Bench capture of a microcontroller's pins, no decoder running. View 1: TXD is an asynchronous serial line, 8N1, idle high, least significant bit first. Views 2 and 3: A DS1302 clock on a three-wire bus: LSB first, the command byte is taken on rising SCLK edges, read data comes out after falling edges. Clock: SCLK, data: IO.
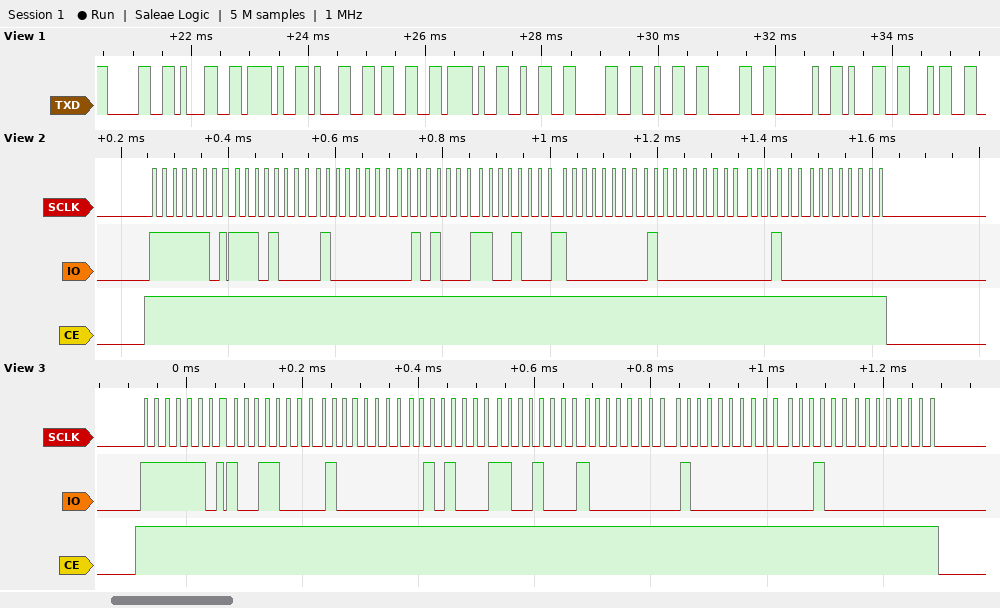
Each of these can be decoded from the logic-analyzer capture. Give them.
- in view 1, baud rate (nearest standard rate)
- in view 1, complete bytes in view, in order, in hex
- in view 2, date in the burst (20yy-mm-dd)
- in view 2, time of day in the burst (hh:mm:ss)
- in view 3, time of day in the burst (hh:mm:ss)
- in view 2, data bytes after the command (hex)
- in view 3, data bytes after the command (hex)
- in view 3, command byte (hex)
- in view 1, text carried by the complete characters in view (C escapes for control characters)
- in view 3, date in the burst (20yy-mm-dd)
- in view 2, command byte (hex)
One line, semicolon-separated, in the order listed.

9600 baud; 30 31 2F 31 33 2F 32 30 32 30 20 31 34; 2020-01-13; 14:02:17; 14:02:19; 17 02 14 13 01 02 20 00; 19 02 14 13 01 02 20 00; 0xBF; "01/13/2020 14"; 2020-01-13; 0xBF
